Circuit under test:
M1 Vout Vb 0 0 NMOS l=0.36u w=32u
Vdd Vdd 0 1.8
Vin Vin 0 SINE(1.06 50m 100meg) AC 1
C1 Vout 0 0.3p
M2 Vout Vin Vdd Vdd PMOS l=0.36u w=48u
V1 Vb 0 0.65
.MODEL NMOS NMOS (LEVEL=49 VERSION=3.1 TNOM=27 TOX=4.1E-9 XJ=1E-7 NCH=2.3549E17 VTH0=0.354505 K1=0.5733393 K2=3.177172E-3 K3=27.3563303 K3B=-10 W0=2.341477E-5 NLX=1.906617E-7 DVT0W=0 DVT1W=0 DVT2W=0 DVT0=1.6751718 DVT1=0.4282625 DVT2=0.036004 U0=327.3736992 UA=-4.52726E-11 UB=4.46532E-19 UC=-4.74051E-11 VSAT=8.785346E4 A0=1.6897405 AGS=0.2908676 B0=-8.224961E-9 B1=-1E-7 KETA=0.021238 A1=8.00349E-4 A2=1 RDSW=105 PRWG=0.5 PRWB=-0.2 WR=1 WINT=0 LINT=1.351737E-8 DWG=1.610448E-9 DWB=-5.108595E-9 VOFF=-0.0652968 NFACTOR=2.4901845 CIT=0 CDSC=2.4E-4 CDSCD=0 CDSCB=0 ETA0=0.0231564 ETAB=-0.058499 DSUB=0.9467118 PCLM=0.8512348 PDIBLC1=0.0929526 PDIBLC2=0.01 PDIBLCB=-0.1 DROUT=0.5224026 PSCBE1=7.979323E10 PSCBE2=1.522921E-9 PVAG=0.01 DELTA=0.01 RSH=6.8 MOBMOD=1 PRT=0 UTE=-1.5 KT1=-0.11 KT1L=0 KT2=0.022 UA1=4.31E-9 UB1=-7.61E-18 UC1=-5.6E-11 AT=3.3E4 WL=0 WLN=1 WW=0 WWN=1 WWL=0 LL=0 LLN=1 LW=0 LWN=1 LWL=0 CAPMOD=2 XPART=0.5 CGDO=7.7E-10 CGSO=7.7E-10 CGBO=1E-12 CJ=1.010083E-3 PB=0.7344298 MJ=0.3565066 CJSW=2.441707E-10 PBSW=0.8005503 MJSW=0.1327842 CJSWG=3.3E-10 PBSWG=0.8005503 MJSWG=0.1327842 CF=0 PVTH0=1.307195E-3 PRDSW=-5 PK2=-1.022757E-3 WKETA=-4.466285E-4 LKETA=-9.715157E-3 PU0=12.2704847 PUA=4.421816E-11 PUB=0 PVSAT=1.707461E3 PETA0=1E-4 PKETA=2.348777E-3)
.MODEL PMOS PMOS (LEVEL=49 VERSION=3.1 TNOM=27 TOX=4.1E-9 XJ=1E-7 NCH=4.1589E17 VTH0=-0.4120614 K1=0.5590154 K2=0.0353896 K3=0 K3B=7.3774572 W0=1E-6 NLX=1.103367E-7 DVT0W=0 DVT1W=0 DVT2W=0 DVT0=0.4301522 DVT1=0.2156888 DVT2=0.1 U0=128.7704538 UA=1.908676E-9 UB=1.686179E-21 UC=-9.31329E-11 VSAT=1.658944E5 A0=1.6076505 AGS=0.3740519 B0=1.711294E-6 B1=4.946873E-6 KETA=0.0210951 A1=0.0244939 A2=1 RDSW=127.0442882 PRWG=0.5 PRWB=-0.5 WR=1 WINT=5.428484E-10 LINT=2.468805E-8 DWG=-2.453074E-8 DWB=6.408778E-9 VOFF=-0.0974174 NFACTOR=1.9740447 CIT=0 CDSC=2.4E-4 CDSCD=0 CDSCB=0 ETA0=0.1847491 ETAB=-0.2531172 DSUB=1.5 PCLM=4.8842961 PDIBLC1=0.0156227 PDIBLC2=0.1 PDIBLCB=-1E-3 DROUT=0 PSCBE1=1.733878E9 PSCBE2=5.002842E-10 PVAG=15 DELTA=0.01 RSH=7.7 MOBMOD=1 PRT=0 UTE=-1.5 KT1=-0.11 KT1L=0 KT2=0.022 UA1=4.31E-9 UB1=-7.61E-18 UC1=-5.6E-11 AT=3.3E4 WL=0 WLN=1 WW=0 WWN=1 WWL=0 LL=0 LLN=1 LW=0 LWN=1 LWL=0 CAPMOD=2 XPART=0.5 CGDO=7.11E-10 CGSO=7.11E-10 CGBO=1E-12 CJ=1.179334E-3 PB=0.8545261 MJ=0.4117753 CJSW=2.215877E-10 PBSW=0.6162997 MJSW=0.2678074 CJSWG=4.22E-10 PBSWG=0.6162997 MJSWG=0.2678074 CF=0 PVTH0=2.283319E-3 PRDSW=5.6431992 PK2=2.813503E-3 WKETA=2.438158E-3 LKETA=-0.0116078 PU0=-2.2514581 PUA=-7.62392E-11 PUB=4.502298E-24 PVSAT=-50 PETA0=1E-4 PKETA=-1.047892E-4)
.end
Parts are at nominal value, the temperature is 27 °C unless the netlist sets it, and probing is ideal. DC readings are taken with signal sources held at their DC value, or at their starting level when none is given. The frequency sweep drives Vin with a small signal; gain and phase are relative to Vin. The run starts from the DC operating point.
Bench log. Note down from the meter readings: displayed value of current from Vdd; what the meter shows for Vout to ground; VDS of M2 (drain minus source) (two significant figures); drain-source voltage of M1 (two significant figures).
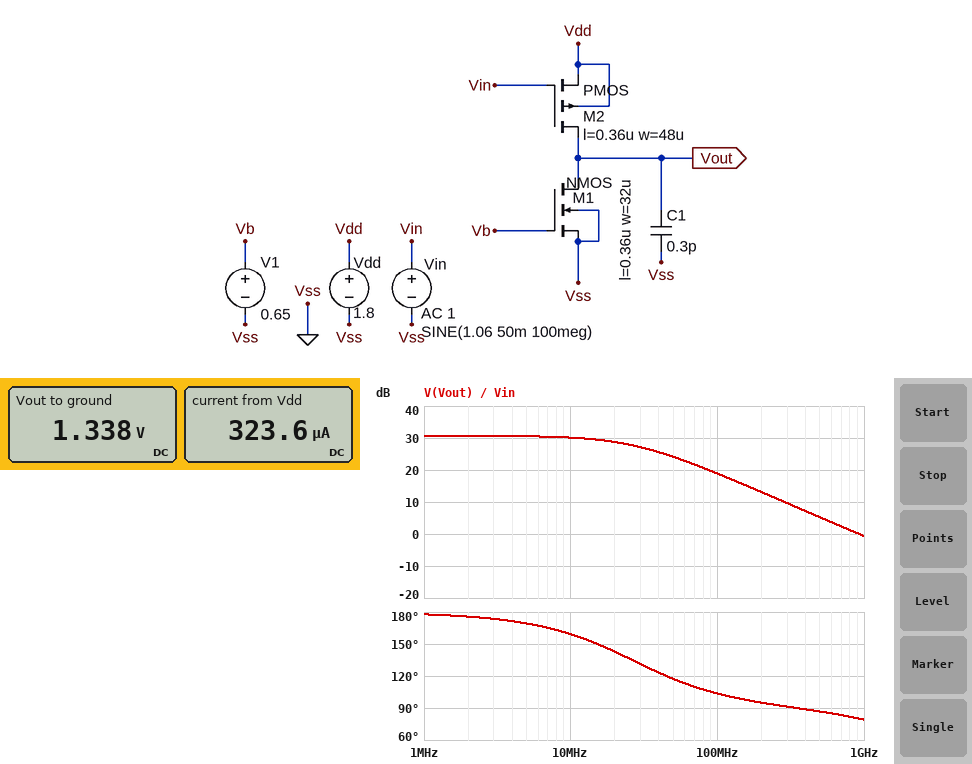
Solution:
323.6 µA
1.338 V
-460 mV
1.3 V
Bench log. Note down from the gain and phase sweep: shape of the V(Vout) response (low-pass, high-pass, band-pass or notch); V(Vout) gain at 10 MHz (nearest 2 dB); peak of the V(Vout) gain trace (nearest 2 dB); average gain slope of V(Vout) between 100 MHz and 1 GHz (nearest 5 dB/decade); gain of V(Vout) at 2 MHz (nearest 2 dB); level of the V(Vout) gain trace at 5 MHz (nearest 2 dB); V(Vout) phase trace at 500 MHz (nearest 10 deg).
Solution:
low-pass
30 dB
30 dB
-20 dB/decade
30 dB
30 dB
90 deg
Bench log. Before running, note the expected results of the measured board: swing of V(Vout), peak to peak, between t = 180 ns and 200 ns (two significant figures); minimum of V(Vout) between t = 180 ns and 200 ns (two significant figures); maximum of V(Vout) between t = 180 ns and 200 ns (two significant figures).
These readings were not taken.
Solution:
800 mV
830 mV
1.6 V
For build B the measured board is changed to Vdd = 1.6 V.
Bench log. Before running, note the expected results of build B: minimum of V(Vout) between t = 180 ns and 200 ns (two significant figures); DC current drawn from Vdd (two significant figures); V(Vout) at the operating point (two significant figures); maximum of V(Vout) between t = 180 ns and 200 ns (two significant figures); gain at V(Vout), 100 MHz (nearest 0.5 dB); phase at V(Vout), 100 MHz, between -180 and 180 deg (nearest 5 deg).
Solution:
4.2 mV
38 µA
11 mV
26 mV
-14.0 dB
170 deg
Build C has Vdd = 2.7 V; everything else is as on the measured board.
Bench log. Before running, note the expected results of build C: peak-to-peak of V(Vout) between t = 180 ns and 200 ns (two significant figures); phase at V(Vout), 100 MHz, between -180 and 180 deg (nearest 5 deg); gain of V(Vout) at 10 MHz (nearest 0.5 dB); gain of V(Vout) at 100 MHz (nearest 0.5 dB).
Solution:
2.6 mV
160 deg
-32.0 dB
-31.5 dB
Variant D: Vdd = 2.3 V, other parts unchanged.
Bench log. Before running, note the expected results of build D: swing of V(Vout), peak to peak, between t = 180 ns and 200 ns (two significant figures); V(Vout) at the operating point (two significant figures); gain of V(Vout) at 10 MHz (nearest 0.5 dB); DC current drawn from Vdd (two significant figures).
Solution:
6.3 mV
2.2 V
-24.0 dB
350 µA
